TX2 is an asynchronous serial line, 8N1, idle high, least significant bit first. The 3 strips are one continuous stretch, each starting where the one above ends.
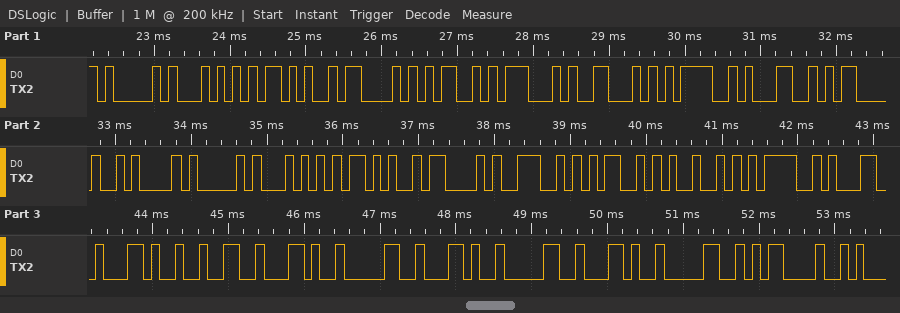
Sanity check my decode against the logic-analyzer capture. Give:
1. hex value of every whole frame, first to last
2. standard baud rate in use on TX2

0x41 0x54 0x2B 0x43 0x4D 0x47 0x46 0x3D 0x31 0x0D 0x0A 0x41 0x54 0x2B 0x43 0x4E 0x4D 0x49 0x3D 0x31 0x2C 0x32 0x2C 0x30 0x2C 0x30 0x2C 0x30 0x0D
9600 baud
